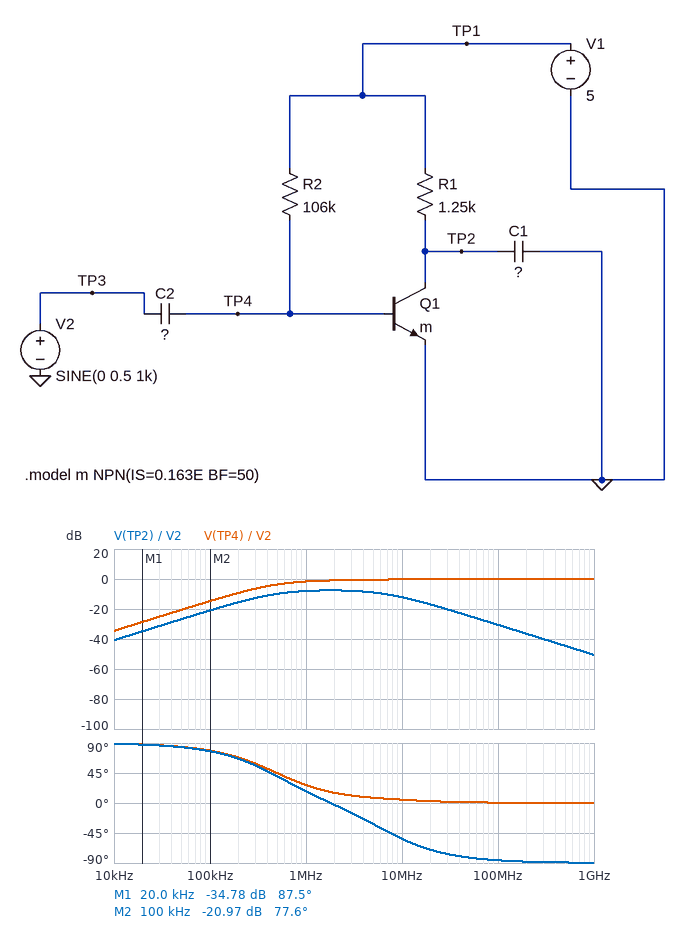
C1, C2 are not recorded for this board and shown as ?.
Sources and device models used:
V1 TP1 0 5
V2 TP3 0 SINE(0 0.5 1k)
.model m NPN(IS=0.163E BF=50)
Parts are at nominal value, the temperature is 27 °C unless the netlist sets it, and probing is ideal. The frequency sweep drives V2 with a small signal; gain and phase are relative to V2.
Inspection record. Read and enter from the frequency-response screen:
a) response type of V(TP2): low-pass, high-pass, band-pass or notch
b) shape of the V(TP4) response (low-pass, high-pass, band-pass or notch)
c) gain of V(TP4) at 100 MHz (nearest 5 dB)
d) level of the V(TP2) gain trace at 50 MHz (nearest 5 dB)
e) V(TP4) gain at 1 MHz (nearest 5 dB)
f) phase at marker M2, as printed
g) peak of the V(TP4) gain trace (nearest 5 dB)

band-pass
high-pass
0 dB
-25 dB
0 dB
77.6 deg
0 dB
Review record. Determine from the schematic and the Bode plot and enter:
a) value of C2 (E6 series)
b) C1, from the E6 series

1 µF
330 nF
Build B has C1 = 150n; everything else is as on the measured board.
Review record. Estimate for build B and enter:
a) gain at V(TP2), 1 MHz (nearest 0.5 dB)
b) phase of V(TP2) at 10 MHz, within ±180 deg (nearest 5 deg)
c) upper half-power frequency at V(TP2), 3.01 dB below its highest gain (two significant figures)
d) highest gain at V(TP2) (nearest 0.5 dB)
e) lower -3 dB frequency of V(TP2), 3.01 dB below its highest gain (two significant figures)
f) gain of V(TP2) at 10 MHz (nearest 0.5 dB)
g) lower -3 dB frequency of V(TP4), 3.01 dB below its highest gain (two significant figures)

-7.5 dB
-35 deg
15 MHz
-7.0 dB
480 kHz
-8.5 dB
560 kHz
